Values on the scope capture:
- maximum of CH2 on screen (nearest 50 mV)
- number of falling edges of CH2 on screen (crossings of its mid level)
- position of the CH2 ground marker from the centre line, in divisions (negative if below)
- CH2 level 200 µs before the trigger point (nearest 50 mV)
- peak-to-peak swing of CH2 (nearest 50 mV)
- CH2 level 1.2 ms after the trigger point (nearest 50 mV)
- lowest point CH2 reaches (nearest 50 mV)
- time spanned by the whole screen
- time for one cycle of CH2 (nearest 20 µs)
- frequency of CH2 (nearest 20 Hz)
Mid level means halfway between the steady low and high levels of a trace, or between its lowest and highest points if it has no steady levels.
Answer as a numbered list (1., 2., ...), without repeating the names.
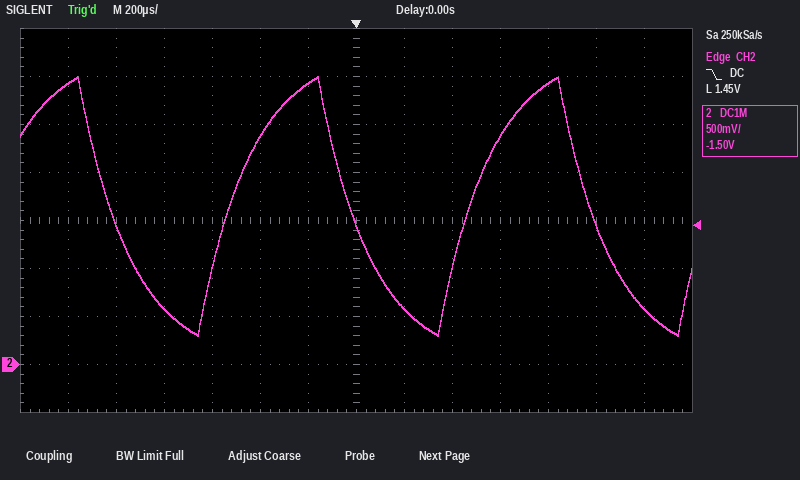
1. 3.00 V
2. 3
3. -3.0 div
4. 2.95 V
5. 2.70 V
6. 600 mV
7. 300 mV
8. 2.8 ms
9. 1.00 ms
10. 1.00 kHz
